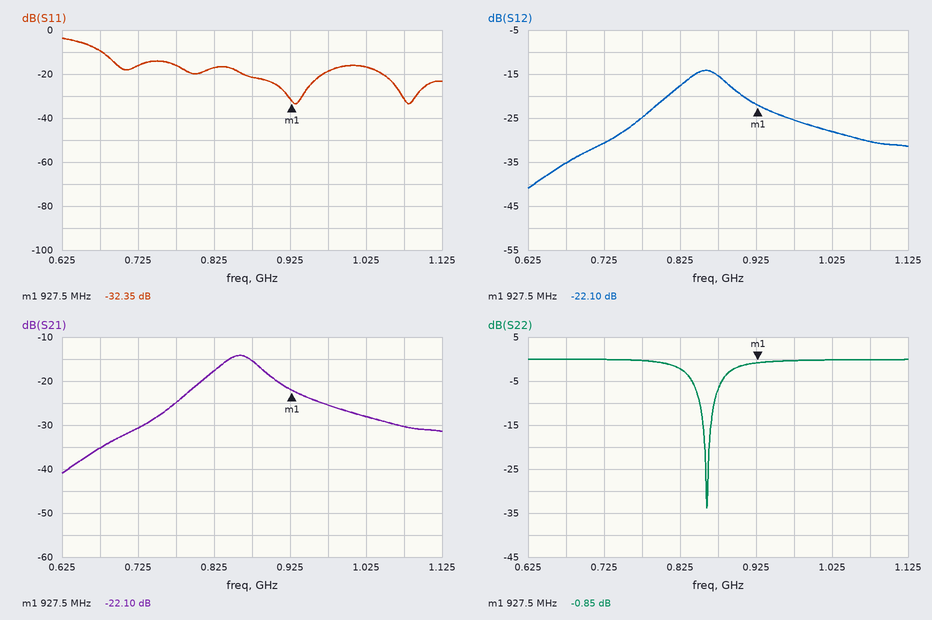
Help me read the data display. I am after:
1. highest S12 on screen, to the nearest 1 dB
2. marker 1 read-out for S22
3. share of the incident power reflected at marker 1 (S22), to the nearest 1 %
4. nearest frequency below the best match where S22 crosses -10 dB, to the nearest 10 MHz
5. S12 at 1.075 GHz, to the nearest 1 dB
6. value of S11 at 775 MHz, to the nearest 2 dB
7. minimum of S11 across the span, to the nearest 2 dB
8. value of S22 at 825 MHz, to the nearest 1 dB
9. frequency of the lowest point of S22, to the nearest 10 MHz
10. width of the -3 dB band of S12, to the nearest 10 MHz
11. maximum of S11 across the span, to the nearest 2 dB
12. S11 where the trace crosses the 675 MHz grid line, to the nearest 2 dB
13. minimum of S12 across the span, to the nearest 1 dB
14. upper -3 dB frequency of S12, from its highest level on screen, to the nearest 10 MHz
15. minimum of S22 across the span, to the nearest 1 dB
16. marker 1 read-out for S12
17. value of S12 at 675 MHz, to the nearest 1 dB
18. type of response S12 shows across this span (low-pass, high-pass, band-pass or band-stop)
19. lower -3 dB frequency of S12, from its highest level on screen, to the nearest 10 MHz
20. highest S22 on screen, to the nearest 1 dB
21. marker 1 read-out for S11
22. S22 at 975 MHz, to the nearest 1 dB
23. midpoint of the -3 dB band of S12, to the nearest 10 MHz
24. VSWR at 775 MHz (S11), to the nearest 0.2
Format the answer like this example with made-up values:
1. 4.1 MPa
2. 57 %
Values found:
1. -14 dB
2. -0.85 dB
3. 82 %
4. 850 MHz
5. -30 dB
6. -16 dB
7. -34 dB
8. -2 dB
9. 860 MHz
10. 60 MHz
11. -4 dB
12. -10 dB
13. -41 dB
14. 890 MHz
15. -34 dB
16. -22.10 dB
17. -35 dB
18. band-pass
19. 830 MHz
20. 0 dB
21. -32.35 dB
22. 0 dB
23. 860 MHz
24. 1.4
